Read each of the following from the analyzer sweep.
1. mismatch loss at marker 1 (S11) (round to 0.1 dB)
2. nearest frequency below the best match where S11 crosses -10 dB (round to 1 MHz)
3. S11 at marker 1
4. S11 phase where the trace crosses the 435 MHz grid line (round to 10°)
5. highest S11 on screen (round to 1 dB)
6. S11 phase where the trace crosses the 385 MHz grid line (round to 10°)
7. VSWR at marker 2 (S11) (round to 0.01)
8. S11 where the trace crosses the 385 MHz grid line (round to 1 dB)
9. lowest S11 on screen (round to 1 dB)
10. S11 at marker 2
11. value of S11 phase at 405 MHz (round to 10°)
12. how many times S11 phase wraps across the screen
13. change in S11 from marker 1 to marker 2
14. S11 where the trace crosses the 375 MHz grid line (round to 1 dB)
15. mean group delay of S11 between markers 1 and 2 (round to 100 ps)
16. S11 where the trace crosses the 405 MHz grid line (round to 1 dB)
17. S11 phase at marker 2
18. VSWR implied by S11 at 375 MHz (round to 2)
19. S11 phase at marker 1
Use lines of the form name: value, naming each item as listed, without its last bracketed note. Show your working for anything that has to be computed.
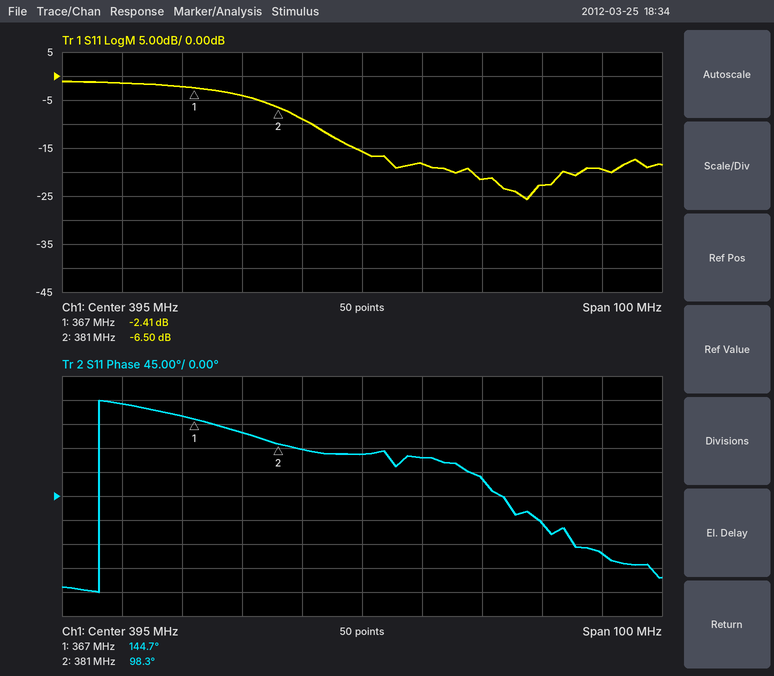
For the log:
mismatch loss at marker 1 (S11): −10 log10(1 − 10^(-2.41/10)) ≈ 3.7 dB
nearest frequency below the best match where S11 crosses -10 dB: 387 MHz
S11 at marker 1: -2.41 dB
S11 phase where the trace crosses the 435 MHz grid line: -110°
highest S11 on screen: -1 dB
S11 phase where the trace crosses the 385 MHz grid line: 90°
VSWR at marker 2 (S11): (1 + 0.4732)/(1 − 0.4732) ≈ 2.80
S11 where the trace crosses the 385 MHz grid line: -9 dB
lowest S11 on screen: -26 dB
S11 at marker 2: -6.50 dB
value of S11 phase at 405 MHz: 70°
how many times S11 phase wraps across the screen: 1
change in S11 from marker 1 to marker 2: -6.5 − (-2.41) = -4.09 dB
S11 where the trace crosses the 375 MHz grid line: -4 dB
mean group delay of S11 between markers 1 and 2: −(98.3° − (144.7°))/(360° × 14 MHz) ≈ 9.2 ns
S11 where the trace crosses the 405 MHz grid line: -18 dB
S11 phase at marker 2: 98.3°
VSWR implied by S11 at 375 MHz: |Γ| = 10^(-4/20) = 0.6310; VSWR = (1 + 0.6310)/(1 − 0.6310) ≈ 4
S11 phase at marker 1: 144.7°
